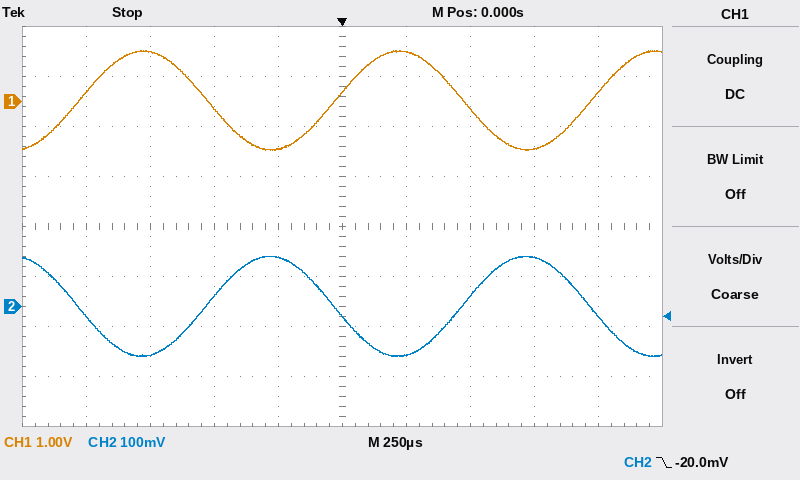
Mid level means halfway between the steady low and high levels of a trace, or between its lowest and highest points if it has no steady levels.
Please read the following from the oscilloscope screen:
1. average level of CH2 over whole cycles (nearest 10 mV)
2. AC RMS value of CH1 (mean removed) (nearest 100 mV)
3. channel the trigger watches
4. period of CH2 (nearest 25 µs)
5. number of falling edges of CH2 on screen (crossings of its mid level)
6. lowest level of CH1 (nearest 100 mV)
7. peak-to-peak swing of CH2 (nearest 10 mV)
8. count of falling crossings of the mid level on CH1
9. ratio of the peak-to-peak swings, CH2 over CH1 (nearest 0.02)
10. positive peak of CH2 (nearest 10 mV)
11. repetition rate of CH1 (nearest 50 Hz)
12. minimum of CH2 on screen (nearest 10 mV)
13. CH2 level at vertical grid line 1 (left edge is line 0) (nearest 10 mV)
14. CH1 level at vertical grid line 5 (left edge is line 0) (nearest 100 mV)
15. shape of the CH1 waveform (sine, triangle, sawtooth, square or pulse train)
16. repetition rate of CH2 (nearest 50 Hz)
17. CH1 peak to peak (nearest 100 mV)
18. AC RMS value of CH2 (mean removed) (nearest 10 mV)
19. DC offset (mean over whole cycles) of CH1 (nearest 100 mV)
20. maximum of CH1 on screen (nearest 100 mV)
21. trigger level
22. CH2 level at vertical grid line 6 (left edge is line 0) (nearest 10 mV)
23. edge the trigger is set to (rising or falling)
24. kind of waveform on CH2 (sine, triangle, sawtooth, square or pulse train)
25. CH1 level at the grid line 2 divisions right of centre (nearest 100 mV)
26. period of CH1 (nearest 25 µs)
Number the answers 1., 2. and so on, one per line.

1. 0 mV
2. 700 mV
3. CH2
4. 1.000 ms
5. 3
6. -1.0 V
7. 200 mV
8. 2
9. 0.10
10. 100 mV
11. 1.00 kHz
12. -100 mV
13. -20 mV
14. 200 mV
15. sine
16. 1.00 kHz
17. 2.0 V
18. 70 mV
19. 0.0 V
20. 1.0 V
21. -20.0 mV
22. -100 mV
23. falling
24. sine
25. -100 mV
26. 1.000 ms
